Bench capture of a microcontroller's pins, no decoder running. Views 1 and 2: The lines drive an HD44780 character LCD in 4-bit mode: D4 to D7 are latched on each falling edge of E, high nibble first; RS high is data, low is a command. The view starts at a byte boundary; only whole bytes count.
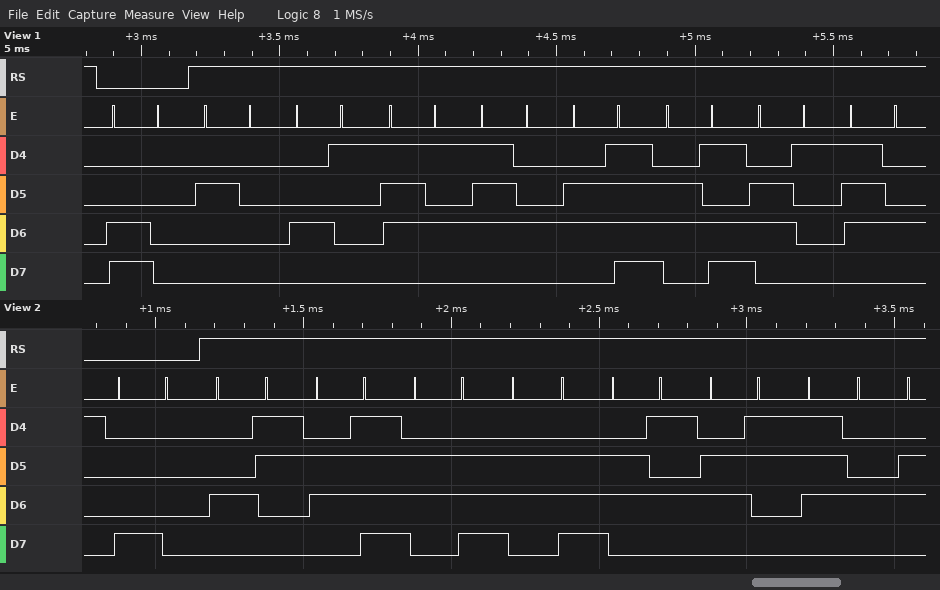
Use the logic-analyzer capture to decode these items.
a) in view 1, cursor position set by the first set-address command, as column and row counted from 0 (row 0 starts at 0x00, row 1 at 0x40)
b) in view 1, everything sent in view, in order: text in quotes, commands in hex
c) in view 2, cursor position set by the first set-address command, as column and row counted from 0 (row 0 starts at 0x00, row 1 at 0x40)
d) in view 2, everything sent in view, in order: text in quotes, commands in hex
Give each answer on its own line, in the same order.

column 0, row 1
0xC0 " Automat"
column 0, row 0
0x80 "Connect"
